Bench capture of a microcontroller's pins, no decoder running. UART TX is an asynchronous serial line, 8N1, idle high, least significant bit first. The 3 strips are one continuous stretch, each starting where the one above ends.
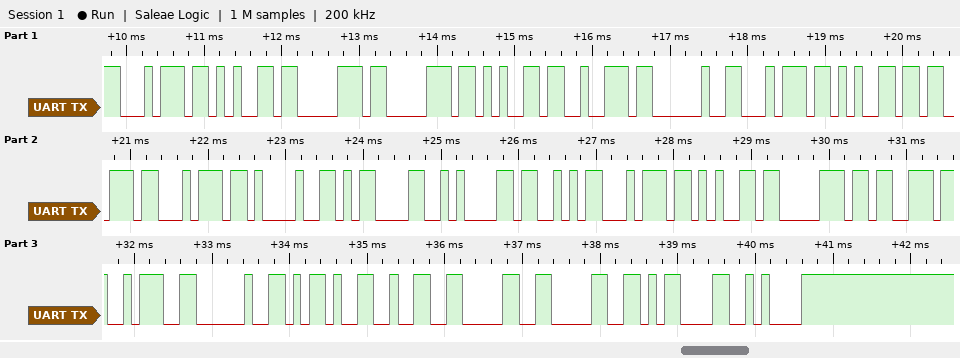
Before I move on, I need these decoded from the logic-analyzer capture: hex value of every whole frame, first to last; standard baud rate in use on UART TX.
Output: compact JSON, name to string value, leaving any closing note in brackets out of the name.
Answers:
{"hex value of every whole frame, first to last": "74 65 70 70 65 72 20 74 65 73 74 21 0D 0A 53 74 65 70 73 3A 20 2D 32 30 30 0D 0A", "standard baud rate in use on UART TX": "9600 baud"}
